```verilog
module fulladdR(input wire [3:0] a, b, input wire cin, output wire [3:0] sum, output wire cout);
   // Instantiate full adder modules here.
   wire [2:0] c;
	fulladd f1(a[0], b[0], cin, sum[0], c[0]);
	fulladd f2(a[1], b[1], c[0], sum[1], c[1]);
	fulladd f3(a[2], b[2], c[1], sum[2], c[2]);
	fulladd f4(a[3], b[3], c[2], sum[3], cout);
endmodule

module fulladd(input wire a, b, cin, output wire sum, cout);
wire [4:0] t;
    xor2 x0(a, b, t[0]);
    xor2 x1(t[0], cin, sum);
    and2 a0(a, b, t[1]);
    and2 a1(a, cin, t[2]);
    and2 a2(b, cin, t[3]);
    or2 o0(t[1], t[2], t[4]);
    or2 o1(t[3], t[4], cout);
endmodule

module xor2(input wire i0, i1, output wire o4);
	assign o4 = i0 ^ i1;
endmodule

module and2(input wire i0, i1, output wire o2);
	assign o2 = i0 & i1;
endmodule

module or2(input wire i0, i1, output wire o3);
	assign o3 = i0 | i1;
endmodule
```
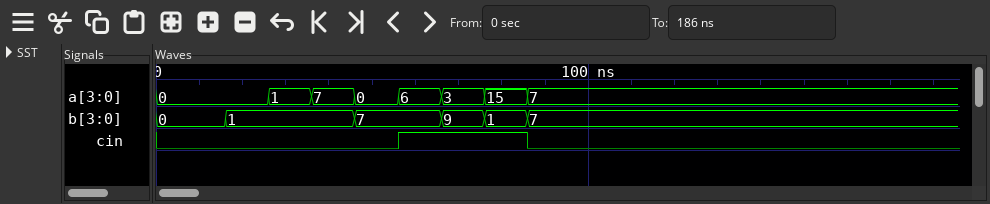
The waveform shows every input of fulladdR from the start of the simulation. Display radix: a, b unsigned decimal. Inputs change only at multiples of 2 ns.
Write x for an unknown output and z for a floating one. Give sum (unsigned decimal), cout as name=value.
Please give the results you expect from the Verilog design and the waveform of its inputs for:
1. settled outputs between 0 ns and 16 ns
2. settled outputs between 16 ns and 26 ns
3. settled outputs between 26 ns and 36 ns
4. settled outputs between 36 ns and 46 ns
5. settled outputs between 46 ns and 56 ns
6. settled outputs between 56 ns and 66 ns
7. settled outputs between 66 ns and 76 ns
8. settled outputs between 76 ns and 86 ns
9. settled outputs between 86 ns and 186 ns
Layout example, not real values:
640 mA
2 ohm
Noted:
sum=0, cout=0
sum=1, cout=0
sum=2, cout=0
sum=8, cout=0
sum=7, cout=0
sum=14, cout=0
sum=13, cout=0
sum=1, cout=1
sum=14, cout=0
